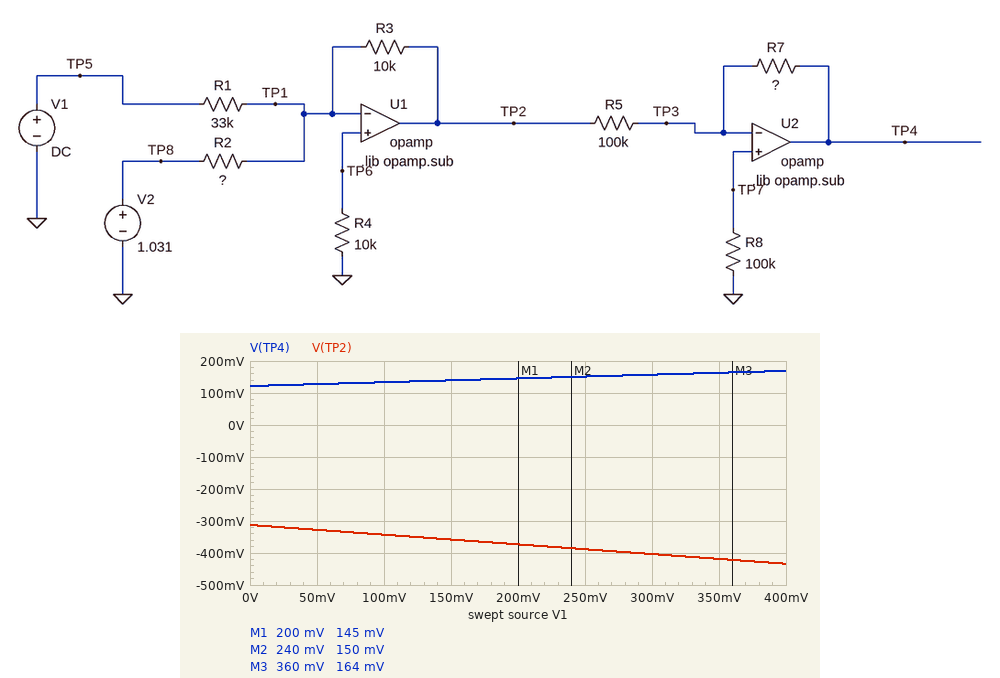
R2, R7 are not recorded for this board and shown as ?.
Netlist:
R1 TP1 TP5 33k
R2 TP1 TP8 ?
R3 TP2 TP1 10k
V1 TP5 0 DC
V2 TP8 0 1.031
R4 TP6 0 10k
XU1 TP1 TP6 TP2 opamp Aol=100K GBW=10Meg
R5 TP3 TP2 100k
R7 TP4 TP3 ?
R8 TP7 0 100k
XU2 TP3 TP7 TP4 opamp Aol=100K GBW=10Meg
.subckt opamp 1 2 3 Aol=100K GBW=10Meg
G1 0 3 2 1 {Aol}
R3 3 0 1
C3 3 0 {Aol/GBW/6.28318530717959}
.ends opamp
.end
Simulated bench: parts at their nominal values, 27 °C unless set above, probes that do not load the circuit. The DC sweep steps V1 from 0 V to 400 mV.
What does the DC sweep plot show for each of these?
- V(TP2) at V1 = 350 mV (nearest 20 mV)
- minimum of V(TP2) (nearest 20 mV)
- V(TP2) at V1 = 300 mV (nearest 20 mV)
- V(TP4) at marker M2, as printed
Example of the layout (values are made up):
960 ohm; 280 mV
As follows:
-420 mV; -440 mV; -400 mV; 150 mV
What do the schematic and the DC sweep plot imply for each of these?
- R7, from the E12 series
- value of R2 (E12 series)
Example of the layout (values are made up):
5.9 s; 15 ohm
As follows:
39 kΩ; 33 kΩ
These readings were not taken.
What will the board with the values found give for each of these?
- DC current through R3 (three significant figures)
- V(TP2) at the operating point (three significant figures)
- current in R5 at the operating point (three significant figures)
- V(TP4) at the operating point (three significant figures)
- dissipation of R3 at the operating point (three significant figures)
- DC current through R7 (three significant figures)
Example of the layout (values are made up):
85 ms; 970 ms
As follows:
31.2 µA; -312 mV; 3.12 µA; 122 mV; 9.76 µW; 3.12 µA
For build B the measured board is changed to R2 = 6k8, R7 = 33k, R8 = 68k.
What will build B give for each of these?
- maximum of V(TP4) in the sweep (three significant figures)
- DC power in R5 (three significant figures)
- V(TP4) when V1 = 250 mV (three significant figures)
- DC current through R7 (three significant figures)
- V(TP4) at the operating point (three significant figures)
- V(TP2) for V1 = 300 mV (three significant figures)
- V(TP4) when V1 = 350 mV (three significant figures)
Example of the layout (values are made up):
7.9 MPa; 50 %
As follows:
540 mV; 23.0 µW; 525 mV; 15.2 µA; 500 mV; -1.61 V; 535 mV
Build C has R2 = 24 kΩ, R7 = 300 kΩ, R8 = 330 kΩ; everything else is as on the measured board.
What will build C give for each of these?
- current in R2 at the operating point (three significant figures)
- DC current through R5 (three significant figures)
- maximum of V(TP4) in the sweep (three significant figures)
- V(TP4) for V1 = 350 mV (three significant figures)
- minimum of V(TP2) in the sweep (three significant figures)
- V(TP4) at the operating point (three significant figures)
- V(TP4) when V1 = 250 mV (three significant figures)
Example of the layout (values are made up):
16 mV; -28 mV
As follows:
43.0 µA; 4.30 µA; 1.65 V; 1.61 V; -551 mV; 1.29 V; 1.52 V
